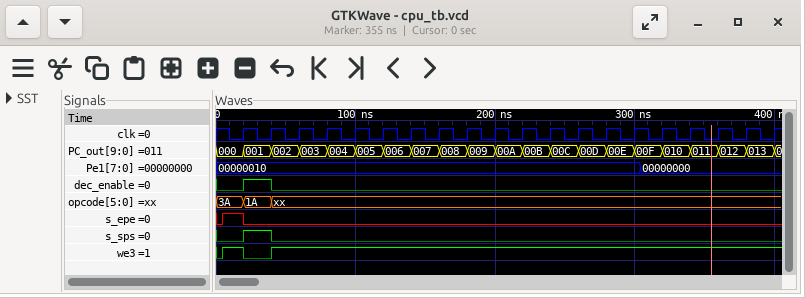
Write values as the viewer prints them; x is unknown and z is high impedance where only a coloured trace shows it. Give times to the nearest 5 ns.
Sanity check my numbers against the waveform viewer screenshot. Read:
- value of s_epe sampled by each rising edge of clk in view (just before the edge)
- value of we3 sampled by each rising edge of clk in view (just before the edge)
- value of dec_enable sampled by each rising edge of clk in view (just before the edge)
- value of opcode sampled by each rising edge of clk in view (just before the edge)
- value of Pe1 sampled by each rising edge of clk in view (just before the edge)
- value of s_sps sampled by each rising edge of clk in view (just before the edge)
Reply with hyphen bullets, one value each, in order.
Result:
- 1 0 0 0 0 0 0 0 0 0 0 0 0 0 0 0 0 0 0 0
- 1 0 1 1 1 1 1 1 1 1 1 1 1 1 1 1 1 1 1 1
- 0 1 0 0 0 0 0 0 0 0 0 0 0 0 0 0 0 0 0 0
- 3A, 1A, xx, xx, xx, xx, xx, xx, xx, xx, xx, xx, xx, xx, xx, xx, xx, xx, xx, xx
- 00000010, 00000010, 00000010, 00000010, 00000010, 00000010, 00000010, 00000010, 00000010, 00000010, 00000010, 00000010, 00000010, 00000010, 00000010, 00000000, 00000000, 00000000, 00000000, 00000000
- 0 1 0 0 0 0 0 0 0 0 0 0 0 0 0 0 0 0 0 0
